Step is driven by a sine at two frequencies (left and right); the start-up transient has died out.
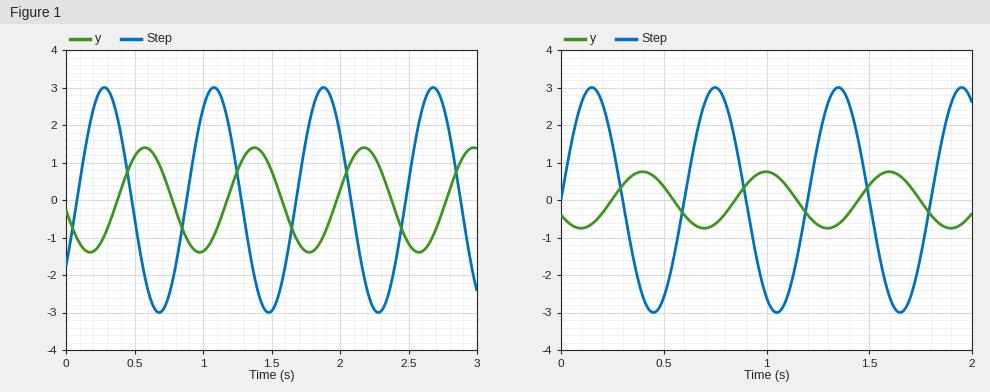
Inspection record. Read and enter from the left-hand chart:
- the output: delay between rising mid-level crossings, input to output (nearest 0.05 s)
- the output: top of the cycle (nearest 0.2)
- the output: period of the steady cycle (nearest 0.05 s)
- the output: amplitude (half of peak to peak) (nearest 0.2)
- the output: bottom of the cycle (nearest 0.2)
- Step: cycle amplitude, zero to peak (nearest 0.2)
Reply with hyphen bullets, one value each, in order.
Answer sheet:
- 0.30 s
- 1.4
- 0.80 s
- 1.4
- -1.4
- 3.0
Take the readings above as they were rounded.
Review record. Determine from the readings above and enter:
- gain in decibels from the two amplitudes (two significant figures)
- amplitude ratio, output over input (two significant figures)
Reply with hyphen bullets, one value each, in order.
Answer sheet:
- -6.6 dB
- 0.47
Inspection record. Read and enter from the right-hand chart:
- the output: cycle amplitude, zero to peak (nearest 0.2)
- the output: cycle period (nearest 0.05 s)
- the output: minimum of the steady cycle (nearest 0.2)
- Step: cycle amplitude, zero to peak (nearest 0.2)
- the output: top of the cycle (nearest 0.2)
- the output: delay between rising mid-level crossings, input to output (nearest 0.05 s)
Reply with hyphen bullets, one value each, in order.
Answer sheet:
- 0.8
- 0.60 s
- -0.8
- 3.0
- 0.8
- 0.25 s
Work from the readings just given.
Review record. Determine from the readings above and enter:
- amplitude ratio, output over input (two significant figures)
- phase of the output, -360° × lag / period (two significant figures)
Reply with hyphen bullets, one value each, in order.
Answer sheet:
- 0.27
- -150°
